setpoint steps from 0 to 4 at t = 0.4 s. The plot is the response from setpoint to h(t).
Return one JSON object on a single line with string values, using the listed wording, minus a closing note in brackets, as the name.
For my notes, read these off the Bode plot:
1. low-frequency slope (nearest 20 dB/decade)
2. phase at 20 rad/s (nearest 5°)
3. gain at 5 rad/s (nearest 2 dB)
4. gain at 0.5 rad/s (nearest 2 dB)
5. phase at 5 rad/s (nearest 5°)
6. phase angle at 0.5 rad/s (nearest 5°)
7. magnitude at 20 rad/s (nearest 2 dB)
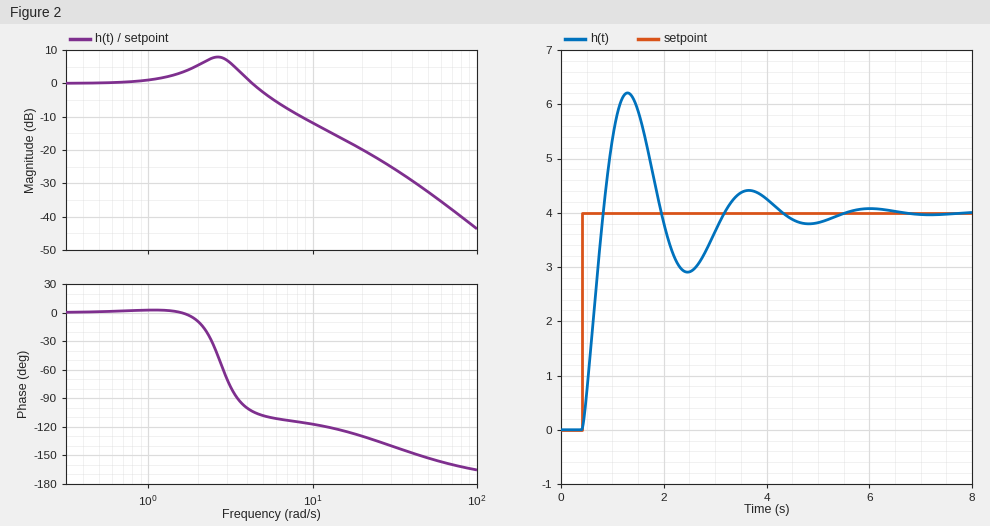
{"low-frequency slope": "0 dB/decade", "phase at 20 rad/s": "-130°", "gain at 5 rad/s": "-2 dB", "gain at 0.5 rad/s": "0 dB", "phase at 5 rad/s": "-110°", "phase angle at 0.5 rad/s": "0°", "magnitude at 20 rad/s": "-20 dB"}
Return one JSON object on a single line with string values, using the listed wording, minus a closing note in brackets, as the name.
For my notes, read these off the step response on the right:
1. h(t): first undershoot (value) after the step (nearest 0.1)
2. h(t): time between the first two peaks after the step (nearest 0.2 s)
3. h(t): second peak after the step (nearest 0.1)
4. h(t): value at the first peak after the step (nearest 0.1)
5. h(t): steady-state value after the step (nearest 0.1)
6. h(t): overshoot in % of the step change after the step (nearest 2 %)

{"h(t): first undershoot (value) after the step": "2.9", "h(t): time between the first two peaks after the step": "2.4 s", "h(t): second peak after the step": "4.4", "h(t): value at the first peak after the step": "6.2", "h(t): steady-state value after the step": "4.0", "h(t): overshoot in % of the step change after the step": "56 %"}
